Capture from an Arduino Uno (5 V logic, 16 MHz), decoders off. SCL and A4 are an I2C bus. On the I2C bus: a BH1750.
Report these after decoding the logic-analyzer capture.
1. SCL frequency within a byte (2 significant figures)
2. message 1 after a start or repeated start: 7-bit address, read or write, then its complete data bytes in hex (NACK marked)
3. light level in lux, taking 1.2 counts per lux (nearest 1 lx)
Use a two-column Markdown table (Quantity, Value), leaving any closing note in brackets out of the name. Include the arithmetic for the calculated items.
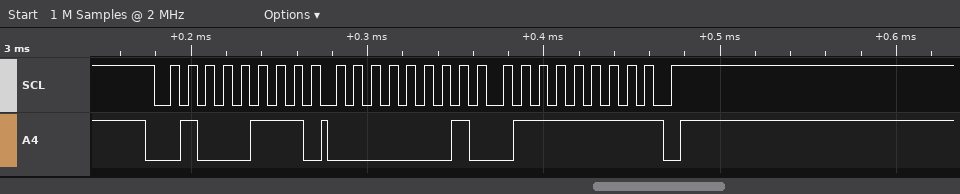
| Quantity | Value |
|---|---|
| SCL frequency within a byte | 100 kHz |
| message 1 after a start or repeated start: 7-bit address, read or write, then its complete data bytes in hex | 0x23 read: 01 7F NACK |
| light level in lux, taking 1.2 counts per lux | 383 / 1.2 = 319 lx |
